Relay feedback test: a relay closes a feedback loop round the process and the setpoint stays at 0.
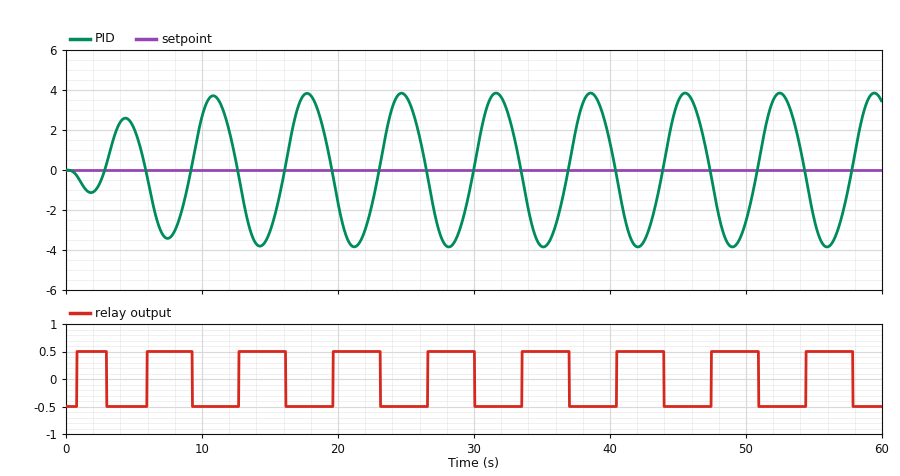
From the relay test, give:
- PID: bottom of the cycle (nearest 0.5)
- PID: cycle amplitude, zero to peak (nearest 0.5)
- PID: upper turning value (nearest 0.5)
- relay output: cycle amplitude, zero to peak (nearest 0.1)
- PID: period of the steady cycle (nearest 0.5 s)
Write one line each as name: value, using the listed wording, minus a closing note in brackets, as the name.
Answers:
PID: bottom of the cycle: -4.0
PID: cycle amplitude, zero to peak: 4.0
PID: upper turning value: 4.0
relay output: cycle amplitude, zero to peak: 0.5
PID: period of the steady cycle: 7.0 s
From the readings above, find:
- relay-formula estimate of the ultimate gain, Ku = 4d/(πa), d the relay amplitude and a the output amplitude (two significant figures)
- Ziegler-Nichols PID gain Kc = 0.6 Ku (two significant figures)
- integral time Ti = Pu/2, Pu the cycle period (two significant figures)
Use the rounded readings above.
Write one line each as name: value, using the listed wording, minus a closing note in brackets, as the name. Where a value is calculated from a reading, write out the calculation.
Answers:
relay-formula estimate of the ultimate gain, Ku = 4d/(πa), d the relay amplitude and a the output amplitude: 4 × 0.5 / (π × 4) = 0.16
Ziegler-Nichols PID gain Kc = 0.6 Ku: 0.6 × 0.16 = 0.096
integral time Ti = Pu/2, Pu the cycle period: 7 / 2 = 3.5 s
